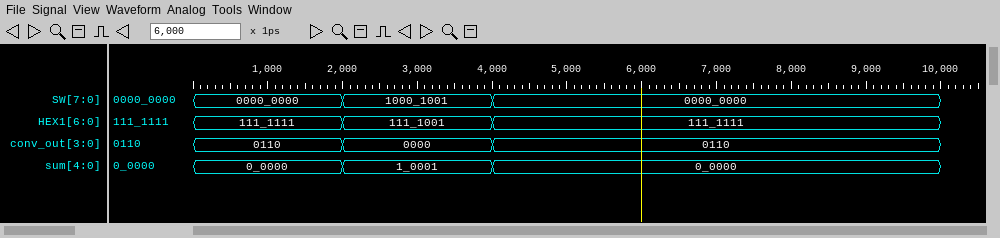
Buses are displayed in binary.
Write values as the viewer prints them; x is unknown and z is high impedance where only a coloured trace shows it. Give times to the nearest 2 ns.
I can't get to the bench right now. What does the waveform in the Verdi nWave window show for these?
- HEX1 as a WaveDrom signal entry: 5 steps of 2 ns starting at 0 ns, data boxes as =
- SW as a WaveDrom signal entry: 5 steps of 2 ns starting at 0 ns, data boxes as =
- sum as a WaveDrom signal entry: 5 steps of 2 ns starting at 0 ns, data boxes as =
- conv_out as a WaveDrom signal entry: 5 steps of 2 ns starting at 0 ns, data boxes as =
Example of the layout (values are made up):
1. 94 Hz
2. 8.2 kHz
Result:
1. {name: 'HEX1', wave: '===..', data: '111_1111 111_1001 111_1111'}
2. {name: 'SW', wave: '===..', data: '0000_0000 1000_1001 0000_0000'}
3. {name: 'sum', wave: '===..', data: '0_0000 1_0001 0_0000'}
4. {name: 'conv_out', wave: '===..', data: '0110 0000 0110'}
